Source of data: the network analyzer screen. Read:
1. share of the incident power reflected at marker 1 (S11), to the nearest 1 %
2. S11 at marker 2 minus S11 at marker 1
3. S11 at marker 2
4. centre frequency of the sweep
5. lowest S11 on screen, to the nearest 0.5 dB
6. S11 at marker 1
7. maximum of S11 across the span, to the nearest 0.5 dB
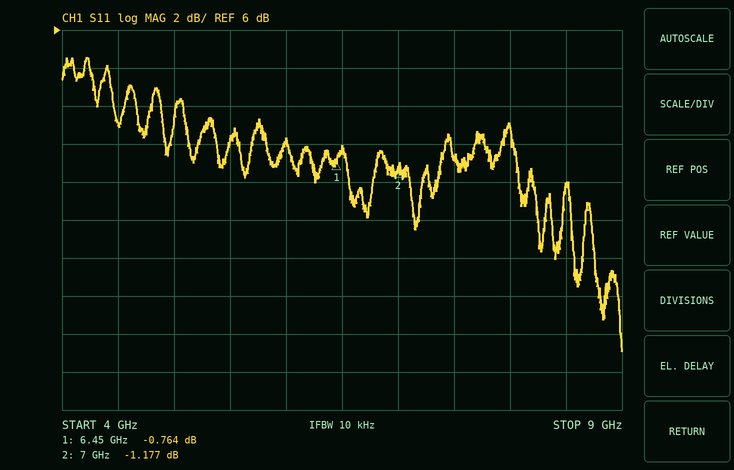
84 %
-0.413 dB
-1.177 dB
6.5 GHz
-11.0 dB
-0.764 dB
4.5 dB
